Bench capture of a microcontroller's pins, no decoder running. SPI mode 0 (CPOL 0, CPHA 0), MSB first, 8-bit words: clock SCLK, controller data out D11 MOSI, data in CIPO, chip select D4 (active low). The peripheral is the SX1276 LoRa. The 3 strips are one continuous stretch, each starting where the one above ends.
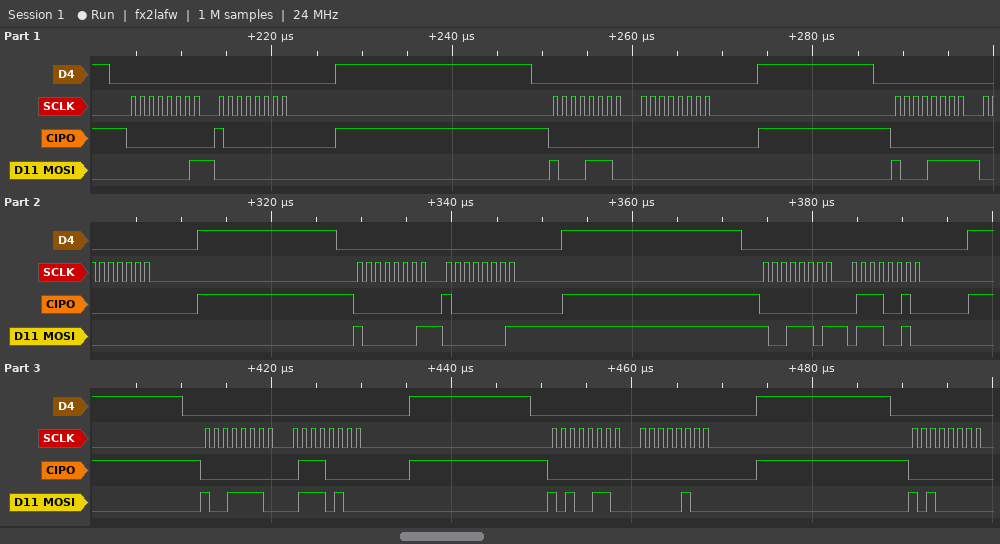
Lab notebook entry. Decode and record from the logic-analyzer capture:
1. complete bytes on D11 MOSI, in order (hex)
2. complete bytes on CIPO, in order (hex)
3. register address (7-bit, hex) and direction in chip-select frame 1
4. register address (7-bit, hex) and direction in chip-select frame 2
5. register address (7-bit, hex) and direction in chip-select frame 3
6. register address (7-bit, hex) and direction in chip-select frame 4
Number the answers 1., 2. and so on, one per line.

1. 0x01 0x00 0x8E 0x00 0x8F 0x00 0x81 0x01 0x9D 0x72 0x9E 0x74 0xA6 0x04 0xA0
2. 0x00 0x80 0x00 0x00 0x00 0x00 0x00 0x80 0x00 0x72 0x00 0x70 0x00 0x00 0x00
3. 0x01 read
4. 0x0E write
5. 0x0F write
6. 0x01 write
